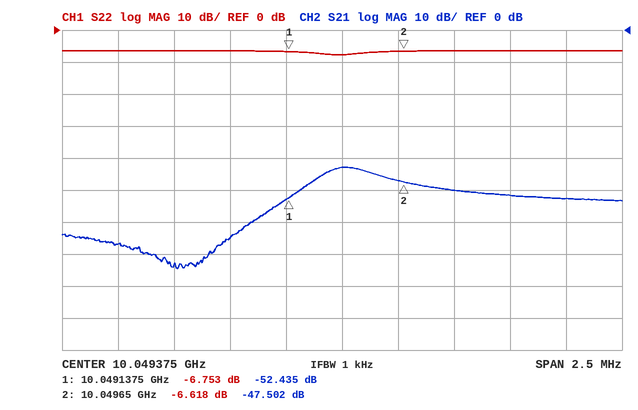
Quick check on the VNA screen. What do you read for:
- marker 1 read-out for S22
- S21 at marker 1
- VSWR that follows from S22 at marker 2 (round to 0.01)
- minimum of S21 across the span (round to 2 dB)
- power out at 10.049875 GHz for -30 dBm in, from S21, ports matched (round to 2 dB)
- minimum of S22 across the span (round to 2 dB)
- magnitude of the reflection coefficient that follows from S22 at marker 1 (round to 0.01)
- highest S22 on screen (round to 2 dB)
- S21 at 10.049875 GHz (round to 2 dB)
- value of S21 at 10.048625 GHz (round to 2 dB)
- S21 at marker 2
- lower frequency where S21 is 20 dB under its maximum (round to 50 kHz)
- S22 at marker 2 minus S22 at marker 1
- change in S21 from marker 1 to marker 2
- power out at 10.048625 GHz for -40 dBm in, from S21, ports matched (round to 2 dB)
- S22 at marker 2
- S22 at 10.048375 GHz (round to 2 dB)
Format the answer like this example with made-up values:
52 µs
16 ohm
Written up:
-6.753 dB
-52.435 dB
2.75
-74 dB
-80 dBm
-8 dB
0.46
-6 dB
-50 dB
-74 dB
-47.502 dB
10.04890 GHz
0.135 dB
4.933 dB
-114 dBm
-6.618 dB
-6 dB
